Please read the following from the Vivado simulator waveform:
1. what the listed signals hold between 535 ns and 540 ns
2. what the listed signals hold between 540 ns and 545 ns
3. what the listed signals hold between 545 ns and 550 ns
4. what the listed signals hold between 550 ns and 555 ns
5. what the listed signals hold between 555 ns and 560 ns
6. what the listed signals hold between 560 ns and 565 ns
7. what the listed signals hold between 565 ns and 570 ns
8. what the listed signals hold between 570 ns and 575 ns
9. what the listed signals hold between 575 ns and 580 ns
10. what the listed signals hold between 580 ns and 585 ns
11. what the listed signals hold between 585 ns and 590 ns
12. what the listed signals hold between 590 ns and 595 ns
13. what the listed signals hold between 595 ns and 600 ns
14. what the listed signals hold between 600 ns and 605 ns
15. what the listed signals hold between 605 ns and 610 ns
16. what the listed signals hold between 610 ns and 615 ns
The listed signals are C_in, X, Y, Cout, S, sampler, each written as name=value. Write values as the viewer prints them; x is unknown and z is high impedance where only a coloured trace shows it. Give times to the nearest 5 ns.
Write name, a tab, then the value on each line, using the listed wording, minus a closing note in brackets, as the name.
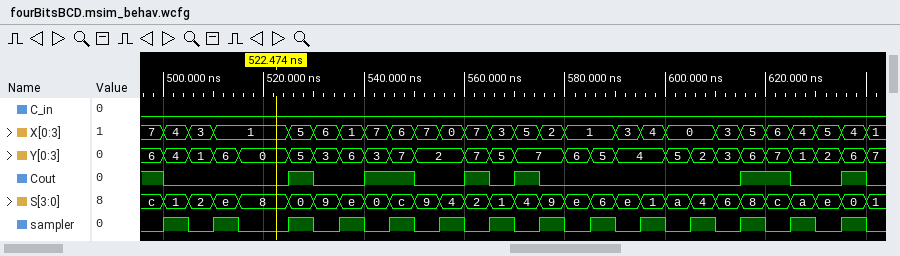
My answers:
what the listed signals hold between 535 ns and 540 ns	C_in=0, X=1, Y=6, Cout=0, S=e, sampler=1
what the listed signals hold between 540 ns and 545 ns	C_in=0, X=7, Y=3, Cout=1, S=0, sampler=0
what the listed signals hold between 545 ns and 550 ns	C_in=0, X=6, Y=7, Cout=1, S=c, sampler=1
what the listed signals hold between 550 ns and 555 ns	C_in=0, X=7, Y=2, Cout=0, S=9, sampler=0
what the listed signals hold between 555 ns and 560 ns	C_in=0, X=0, Y=2, Cout=0, S=4, sampler=1
what the listed signals hold between 560 ns and 565 ns	C_in=0, X=7, Y=7, Cout=1, S=2, sampler=0
what the listed signals hold between 565 ns and 570 ns	C_in=0, X=3, Y=5, Cout=0, S=1, sampler=1
what the listed signals hold between 570 ns and 575 ns	C_in=0, X=5, Y=7, Cout=1, S=4, sampler=0
what the listed signals hold between 575 ns and 580 ns	C_in=0, X=2, Y=7, Cout=0, S=9, sampler=1
what the listed signals hold between 580 ns and 585 ns	C_in=0, X=1, Y=6, Cout=0, S=e, sampler=0
what the listed signals hold between 585 ns and 590 ns	C_in=0, X=1, Y=5, Cout=0, S=6, sampler=1
what the listed signals hold between 590 ns and 595 ns	C_in=0, X=3, Y=4, Cout=0, S=e, sampler=0
what the listed signals hold between 595 ns and 600 ns	C_in=0, X=4, Y=4, Cout=0, S=1, sampler=1
what the listed signals hold between 600 ns and 605 ns	C_in=0, X=0, Y=5, Cout=0, S=a, sampler=0
what the listed signals hold between 605 ns and 610 ns	C_in=0, X=0, Y=2, Cout=0, S=4, sampler=1
what the listed signals hold between 610 ns and 615 ns	C_in=0, X=3, Y=3, Cout=0, S=6, sampler=0
